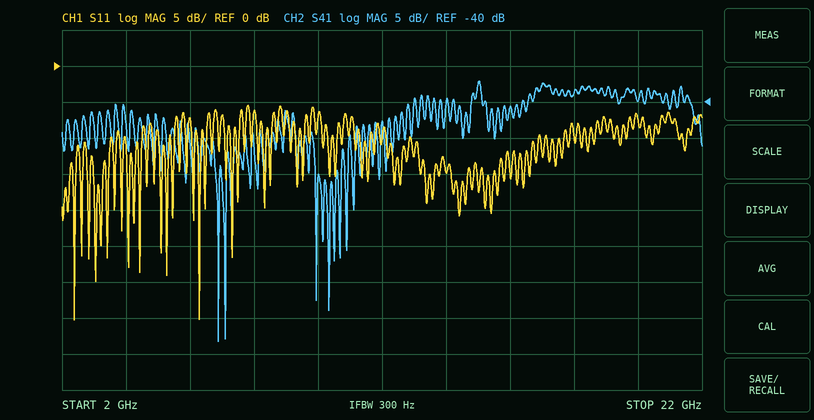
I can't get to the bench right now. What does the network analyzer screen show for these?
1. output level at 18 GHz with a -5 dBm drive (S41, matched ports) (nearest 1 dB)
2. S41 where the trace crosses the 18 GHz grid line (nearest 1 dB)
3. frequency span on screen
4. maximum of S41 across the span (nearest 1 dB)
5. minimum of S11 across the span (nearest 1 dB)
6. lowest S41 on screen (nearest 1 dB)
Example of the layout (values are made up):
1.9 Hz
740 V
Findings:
-44 dBm
-39 dB
20 GHz
-37 dB
-35 dB
-73 dB
